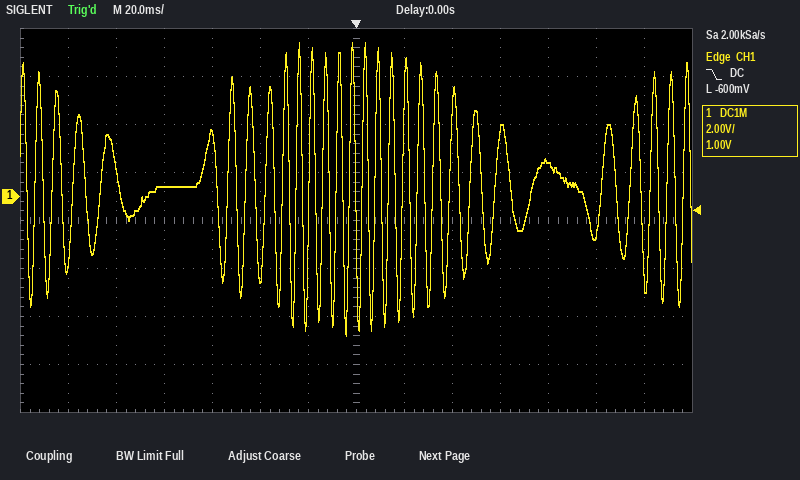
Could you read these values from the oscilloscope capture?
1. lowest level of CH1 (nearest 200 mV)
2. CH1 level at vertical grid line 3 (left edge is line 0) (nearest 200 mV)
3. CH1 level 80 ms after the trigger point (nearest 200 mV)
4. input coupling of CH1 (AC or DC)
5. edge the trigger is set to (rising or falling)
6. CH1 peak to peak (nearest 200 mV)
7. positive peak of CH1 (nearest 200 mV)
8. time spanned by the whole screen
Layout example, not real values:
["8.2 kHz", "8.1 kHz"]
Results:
["-5.8 V", "400 mV", "1.4 V", "DC", "falling", "12.2 V", "6.4 V", "280 ms"]
